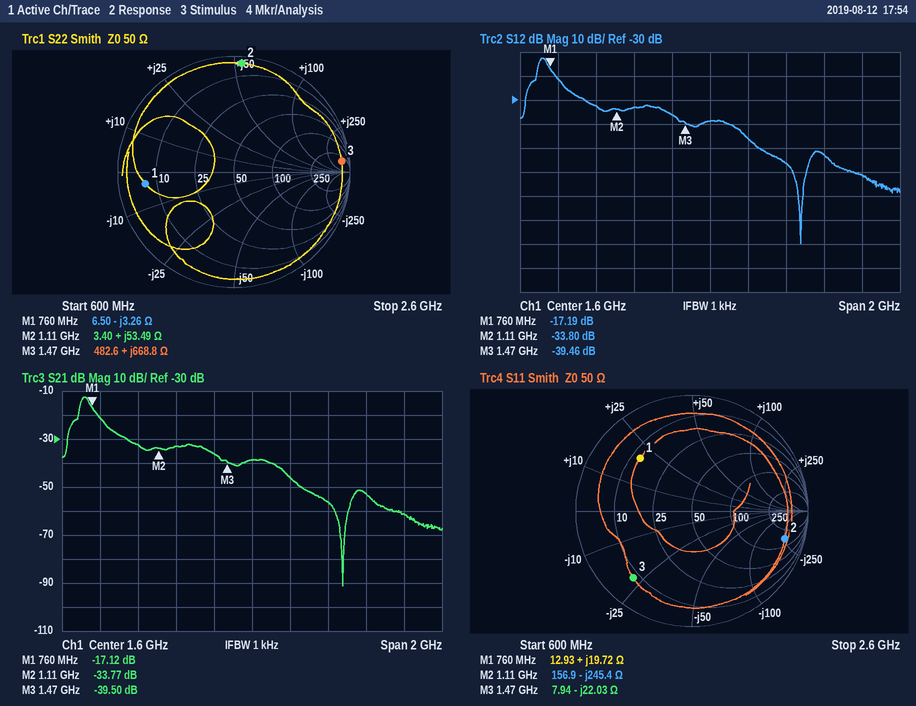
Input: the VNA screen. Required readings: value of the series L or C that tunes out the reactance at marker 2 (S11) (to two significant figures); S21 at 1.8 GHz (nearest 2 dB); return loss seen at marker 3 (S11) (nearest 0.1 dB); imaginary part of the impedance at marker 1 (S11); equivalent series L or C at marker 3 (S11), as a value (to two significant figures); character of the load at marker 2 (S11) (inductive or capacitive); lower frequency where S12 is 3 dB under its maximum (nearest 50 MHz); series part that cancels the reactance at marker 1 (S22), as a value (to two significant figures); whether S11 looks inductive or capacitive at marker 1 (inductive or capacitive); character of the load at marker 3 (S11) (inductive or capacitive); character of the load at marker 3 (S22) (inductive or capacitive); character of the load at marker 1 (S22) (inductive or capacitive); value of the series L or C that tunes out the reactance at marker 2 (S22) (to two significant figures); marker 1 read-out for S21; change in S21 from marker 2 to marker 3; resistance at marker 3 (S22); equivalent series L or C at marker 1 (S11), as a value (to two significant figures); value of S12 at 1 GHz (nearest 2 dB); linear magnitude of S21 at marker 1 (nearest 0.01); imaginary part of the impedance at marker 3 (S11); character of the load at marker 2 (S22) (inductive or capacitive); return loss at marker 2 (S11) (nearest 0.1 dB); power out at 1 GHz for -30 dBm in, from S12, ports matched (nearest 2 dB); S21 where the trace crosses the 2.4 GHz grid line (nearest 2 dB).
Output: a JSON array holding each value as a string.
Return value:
["35 nH", "-46 dB", "2.3 dB", "+19.72 Ω", "4.9 pF", "capacitive", "700 MHz", "680 pH", "inductive", "capacitive", "inductive", "capacitive", "2.7 pF", "-17.12 dB", "-5.73 dB", "482.6 Ω", "4.1 nH", "-32 dB", "0.14", "-22.03 Ω", "inductive", "1.6 dB", "-62 dBm", "-62 dB"]
